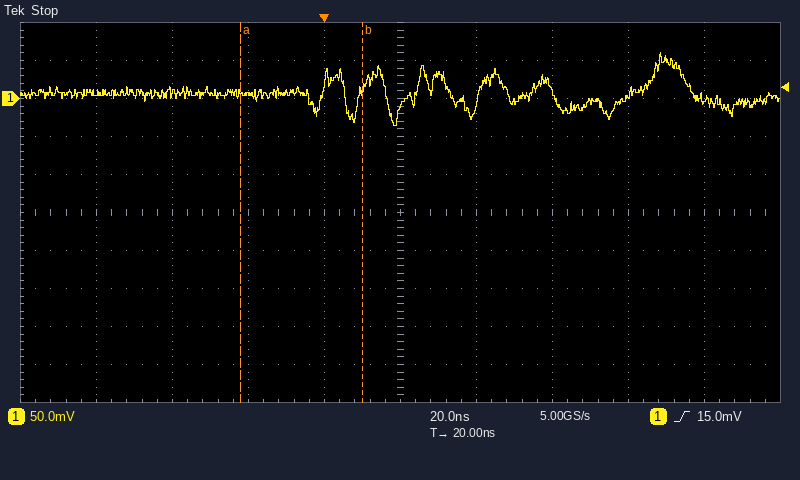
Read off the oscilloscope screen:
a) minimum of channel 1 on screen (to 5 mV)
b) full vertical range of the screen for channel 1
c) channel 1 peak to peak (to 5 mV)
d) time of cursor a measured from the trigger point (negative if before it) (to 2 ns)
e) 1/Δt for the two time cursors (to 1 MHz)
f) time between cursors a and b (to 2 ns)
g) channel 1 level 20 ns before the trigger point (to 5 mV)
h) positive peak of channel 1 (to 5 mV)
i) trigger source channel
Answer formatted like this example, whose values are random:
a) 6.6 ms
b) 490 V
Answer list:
a) -35 mV
b) 500 mV
c) 95 mV
d) -22 ns
e) 31 MHz
f) 32 ns
g) 5 mV
h) 60 mV
i) channel 1
